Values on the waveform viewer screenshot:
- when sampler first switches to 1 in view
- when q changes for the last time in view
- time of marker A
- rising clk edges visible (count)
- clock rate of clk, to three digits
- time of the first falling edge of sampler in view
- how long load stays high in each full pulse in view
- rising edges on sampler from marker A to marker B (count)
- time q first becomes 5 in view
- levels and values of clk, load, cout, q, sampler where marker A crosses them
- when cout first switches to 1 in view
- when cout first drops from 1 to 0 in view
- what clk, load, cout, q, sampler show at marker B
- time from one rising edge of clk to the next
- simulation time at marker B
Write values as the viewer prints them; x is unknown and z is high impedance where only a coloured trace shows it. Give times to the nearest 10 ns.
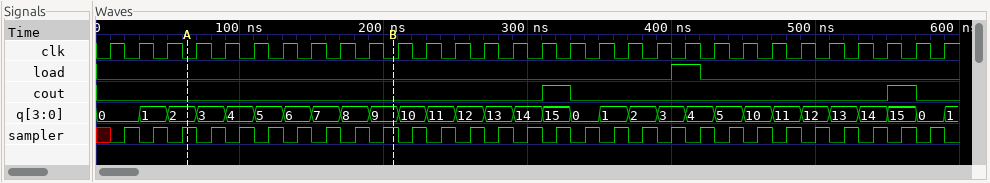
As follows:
20 ns
590 ns
60 ns
30
50.0 MHz
30 ns
20 ns
7
110 ns
clk=0, load=0, cout=0, q=2, sampler=1
310 ns
330 ns
clk=0, load=0, cout=0, q=9, sampler=1
20 ns
210 ns
